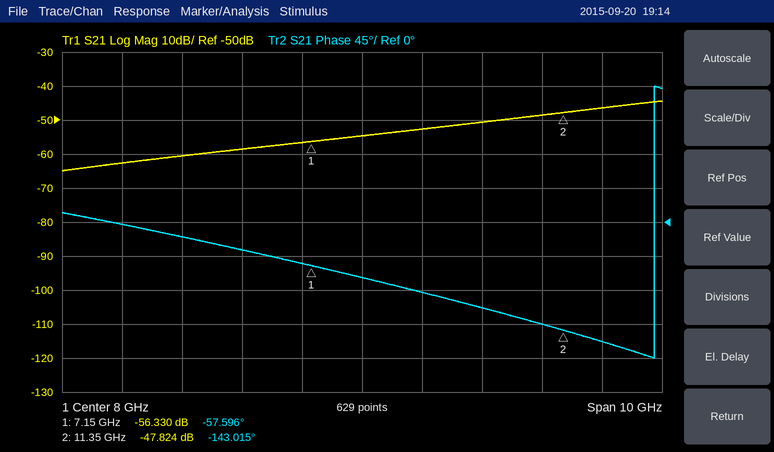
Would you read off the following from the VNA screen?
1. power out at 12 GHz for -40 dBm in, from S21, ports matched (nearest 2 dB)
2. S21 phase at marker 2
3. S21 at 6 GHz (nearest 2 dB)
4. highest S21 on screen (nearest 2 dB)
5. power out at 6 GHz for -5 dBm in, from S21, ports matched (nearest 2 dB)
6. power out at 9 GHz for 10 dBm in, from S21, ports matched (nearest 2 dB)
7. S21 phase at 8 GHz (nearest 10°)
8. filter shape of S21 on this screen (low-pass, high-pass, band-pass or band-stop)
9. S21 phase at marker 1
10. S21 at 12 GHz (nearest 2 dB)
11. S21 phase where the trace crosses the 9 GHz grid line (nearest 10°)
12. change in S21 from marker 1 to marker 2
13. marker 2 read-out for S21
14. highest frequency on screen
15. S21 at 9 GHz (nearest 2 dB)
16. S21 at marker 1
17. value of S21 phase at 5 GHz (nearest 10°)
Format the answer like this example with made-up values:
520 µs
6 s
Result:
-86 dBm
-143.015°
-58 dB
-44 dB
-64 dBm
-42 dBm
-70°
high-pass
-57.596°
-46 dB
-90°
8.506 dB
-47.824 dB
13 GHz
-52 dB
-56.330 dB
-20°
